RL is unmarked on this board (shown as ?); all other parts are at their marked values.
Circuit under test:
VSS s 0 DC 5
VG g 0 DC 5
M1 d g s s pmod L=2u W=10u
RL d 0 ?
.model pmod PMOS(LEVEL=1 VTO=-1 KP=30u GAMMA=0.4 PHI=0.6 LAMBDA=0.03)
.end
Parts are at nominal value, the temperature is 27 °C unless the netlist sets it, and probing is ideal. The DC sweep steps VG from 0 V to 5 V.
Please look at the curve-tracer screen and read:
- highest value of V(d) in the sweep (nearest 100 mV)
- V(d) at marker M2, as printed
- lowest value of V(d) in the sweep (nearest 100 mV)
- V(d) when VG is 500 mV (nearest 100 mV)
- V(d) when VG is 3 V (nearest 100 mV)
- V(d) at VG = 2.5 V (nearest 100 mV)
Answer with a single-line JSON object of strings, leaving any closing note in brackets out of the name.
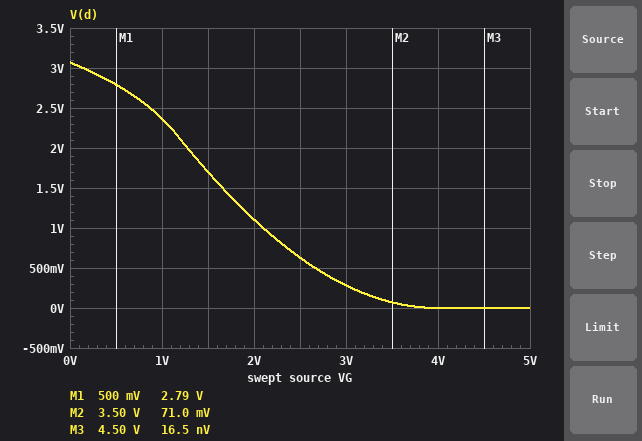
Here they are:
{"highest value of V(d) in the sweep": "3.1 V", "V(d) at marker M2, as printed": "71.0 mV", "lowest value of V(d) in the sweep": "0 V", "V(d) when VG is 500 mV": "2.8 V", "V(d) when VG is 3 V": "300 mV", "V(d) at VG = 2.5 V": "600 mV"}
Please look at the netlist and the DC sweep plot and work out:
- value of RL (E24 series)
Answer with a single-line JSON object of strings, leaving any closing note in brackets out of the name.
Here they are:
{"value of RL": "3.3 kΩ"}
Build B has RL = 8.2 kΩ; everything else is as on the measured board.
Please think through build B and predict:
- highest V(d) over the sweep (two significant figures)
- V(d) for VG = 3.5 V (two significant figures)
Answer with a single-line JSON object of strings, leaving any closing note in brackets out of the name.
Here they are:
{"highest V(d) over the sweep": "4.1 V", "V(d) for VG = 3.5 V": "180 mV"}
